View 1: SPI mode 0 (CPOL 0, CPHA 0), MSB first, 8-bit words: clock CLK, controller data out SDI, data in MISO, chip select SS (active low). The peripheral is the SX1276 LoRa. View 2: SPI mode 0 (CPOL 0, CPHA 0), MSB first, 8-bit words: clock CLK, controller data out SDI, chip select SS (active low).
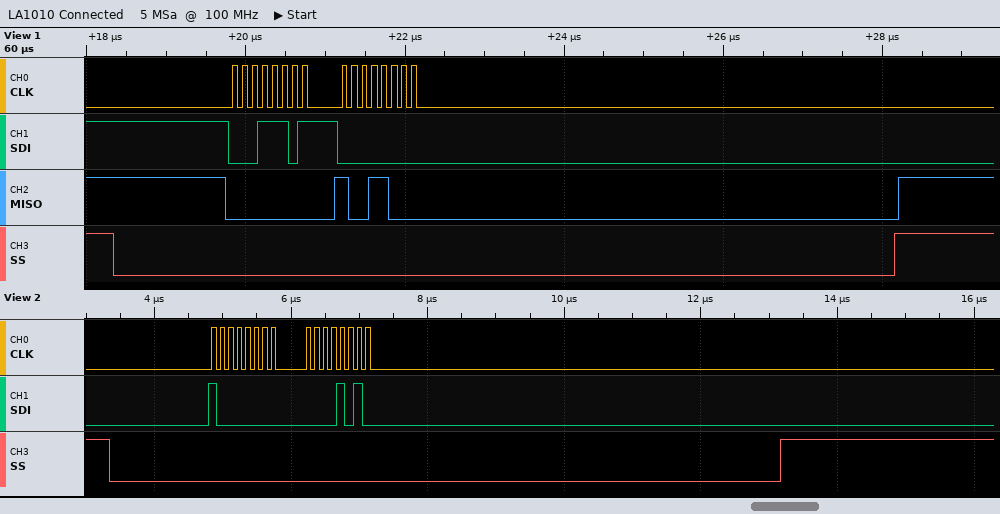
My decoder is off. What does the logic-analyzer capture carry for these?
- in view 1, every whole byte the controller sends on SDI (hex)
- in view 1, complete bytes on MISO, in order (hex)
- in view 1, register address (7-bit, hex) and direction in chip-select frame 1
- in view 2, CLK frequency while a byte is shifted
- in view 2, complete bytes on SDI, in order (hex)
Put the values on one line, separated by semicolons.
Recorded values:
0x1D 0x00; 0x00 0x98; 0x1D read; 8 MHz; 80 0A
